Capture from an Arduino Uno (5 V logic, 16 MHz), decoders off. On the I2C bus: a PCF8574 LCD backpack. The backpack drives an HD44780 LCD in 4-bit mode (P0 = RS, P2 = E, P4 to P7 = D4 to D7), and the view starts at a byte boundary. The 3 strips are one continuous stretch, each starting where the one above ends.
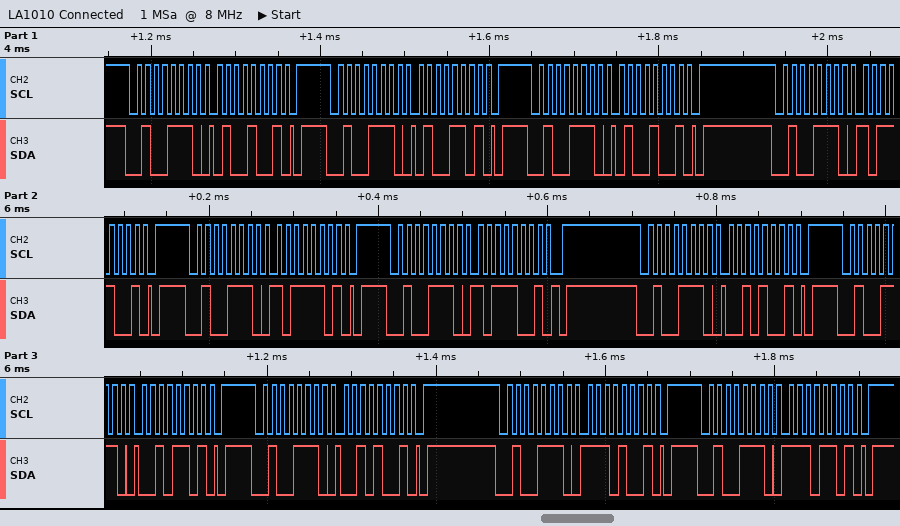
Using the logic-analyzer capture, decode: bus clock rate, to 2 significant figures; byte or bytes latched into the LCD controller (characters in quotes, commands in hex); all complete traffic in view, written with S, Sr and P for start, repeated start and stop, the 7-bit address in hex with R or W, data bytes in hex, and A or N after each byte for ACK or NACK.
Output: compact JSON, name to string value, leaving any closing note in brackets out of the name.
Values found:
{"bus clock rate, to 2 significant figures": "100 kHz", "byte or bytes latched into the LCD controller": "'K'", "all complete traffic in view, written with S, Sr and P for start, repeated start and stop, the 7-bit address in hex with R or W, data bytes in hex, and A or N after each byte for ACK or NACK": "S 27W A 49 A P S 27W A 4D A P S 27W A 49 A P S 27W A B9 A P S 27W A BD A P S 27W A B9 A P S 27W A 29 A P S 27W A 2D A P S 27W A 29 A P S 27W A E9 A P S 27W A ED A P"}
